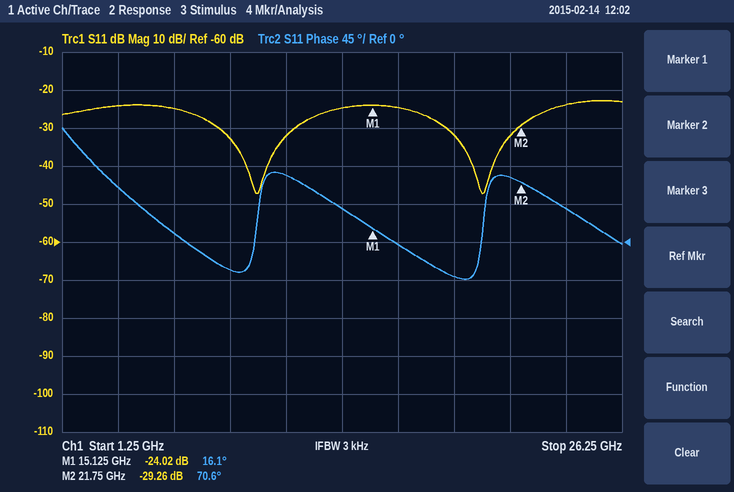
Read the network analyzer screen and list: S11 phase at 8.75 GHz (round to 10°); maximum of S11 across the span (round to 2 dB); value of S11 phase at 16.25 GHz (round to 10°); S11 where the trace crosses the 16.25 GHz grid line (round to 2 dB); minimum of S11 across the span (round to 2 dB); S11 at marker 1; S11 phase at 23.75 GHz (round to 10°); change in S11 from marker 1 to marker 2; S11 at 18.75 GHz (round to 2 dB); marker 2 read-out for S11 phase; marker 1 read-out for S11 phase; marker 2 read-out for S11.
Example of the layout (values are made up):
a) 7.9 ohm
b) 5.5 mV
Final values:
a) -30°
b) -22 dB
c) 0°
d) -24 dB
e) -48 dB
f) -24.02 dB
g) 40°
h) -5.24 dB
i) -32 dB
j) 70.6°
k) 16.1°
l) -29.26 dB
